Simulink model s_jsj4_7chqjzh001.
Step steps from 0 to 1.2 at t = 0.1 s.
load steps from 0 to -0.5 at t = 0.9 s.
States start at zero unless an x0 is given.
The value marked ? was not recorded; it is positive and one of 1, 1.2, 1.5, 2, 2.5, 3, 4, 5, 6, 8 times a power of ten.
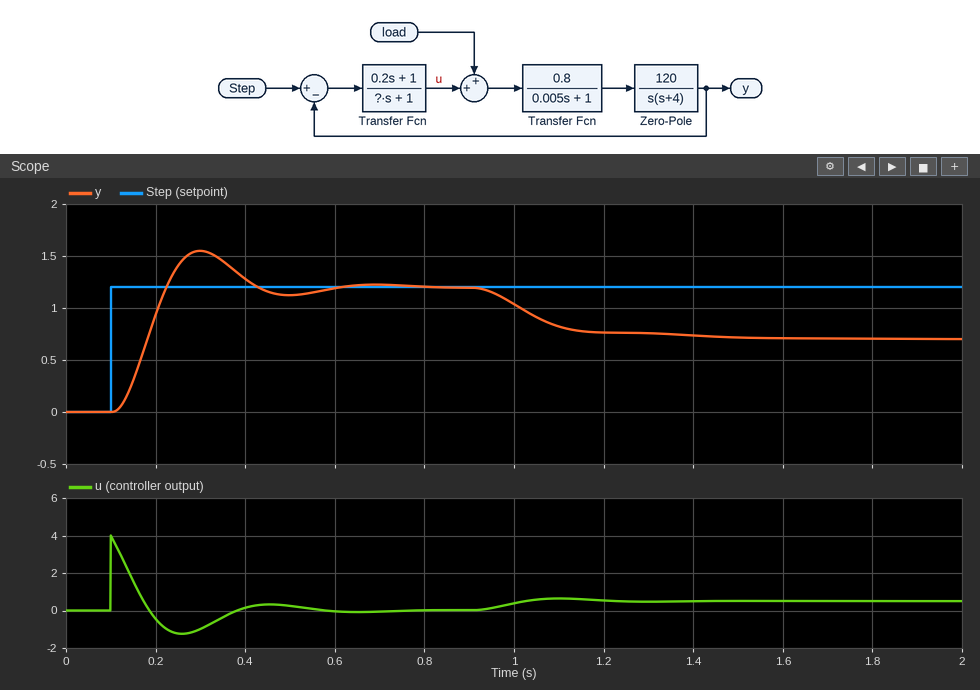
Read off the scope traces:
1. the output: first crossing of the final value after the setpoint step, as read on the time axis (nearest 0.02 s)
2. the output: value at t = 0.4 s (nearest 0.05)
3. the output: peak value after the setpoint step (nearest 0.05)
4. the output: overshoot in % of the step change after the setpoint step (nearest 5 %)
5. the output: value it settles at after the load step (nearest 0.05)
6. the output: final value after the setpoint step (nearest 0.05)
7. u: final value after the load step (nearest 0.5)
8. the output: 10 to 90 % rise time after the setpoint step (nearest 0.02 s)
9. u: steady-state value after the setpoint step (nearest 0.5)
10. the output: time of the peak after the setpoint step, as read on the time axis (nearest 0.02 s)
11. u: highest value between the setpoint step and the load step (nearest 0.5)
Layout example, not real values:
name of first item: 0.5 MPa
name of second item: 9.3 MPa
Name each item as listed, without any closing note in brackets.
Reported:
the output: first crossing of the final value after the setpoint step, as read on the time axis: 0.22 s
the output: value at t = 0.4 s: 1.30
the output: peak value after the setpoint step: 1.55
the output: overshoot in % of the step change after the setpoint step: 30 %
the output: value it settles at after the load step: 0.70
the output: final value after the setpoint step: 1.20
u: final value after the load step: 0.5
the output: 10 to 90 % rise time after the setpoint step: 0.08 s
u: steady-state value after the setpoint step: 0.0
the output: time of the peak after the setpoint step, as read on the time axis: 0.30 s
u: highest value between the setpoint step and the load step: 4.0
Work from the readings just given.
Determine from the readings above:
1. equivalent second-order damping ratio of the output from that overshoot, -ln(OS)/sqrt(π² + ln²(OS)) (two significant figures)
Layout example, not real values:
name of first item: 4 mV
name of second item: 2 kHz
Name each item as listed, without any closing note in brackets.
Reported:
equivalent second-order damping ratio of the output from that overshoot, -ln(OS)/sqrt(π² + ln²(OS)): 0.36
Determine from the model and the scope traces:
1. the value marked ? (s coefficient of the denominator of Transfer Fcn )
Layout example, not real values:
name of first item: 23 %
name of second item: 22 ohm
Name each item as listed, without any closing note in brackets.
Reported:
the value marked ?: 0.06
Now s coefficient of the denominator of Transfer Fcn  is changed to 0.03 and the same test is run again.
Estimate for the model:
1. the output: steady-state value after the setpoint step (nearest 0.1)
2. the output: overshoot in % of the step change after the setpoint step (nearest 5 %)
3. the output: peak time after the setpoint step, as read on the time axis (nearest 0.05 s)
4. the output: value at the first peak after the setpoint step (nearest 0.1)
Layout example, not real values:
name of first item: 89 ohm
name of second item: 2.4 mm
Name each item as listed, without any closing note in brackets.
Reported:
the output: steady-state value after the setpoint step: 1.2
the output: overshoot in % of the step change after the setpoint step: 15 %
the output: peak time after the setpoint step, as read on the time axis: 0.25 s
the output: value at the first peak after the setpoint step: 1.4
